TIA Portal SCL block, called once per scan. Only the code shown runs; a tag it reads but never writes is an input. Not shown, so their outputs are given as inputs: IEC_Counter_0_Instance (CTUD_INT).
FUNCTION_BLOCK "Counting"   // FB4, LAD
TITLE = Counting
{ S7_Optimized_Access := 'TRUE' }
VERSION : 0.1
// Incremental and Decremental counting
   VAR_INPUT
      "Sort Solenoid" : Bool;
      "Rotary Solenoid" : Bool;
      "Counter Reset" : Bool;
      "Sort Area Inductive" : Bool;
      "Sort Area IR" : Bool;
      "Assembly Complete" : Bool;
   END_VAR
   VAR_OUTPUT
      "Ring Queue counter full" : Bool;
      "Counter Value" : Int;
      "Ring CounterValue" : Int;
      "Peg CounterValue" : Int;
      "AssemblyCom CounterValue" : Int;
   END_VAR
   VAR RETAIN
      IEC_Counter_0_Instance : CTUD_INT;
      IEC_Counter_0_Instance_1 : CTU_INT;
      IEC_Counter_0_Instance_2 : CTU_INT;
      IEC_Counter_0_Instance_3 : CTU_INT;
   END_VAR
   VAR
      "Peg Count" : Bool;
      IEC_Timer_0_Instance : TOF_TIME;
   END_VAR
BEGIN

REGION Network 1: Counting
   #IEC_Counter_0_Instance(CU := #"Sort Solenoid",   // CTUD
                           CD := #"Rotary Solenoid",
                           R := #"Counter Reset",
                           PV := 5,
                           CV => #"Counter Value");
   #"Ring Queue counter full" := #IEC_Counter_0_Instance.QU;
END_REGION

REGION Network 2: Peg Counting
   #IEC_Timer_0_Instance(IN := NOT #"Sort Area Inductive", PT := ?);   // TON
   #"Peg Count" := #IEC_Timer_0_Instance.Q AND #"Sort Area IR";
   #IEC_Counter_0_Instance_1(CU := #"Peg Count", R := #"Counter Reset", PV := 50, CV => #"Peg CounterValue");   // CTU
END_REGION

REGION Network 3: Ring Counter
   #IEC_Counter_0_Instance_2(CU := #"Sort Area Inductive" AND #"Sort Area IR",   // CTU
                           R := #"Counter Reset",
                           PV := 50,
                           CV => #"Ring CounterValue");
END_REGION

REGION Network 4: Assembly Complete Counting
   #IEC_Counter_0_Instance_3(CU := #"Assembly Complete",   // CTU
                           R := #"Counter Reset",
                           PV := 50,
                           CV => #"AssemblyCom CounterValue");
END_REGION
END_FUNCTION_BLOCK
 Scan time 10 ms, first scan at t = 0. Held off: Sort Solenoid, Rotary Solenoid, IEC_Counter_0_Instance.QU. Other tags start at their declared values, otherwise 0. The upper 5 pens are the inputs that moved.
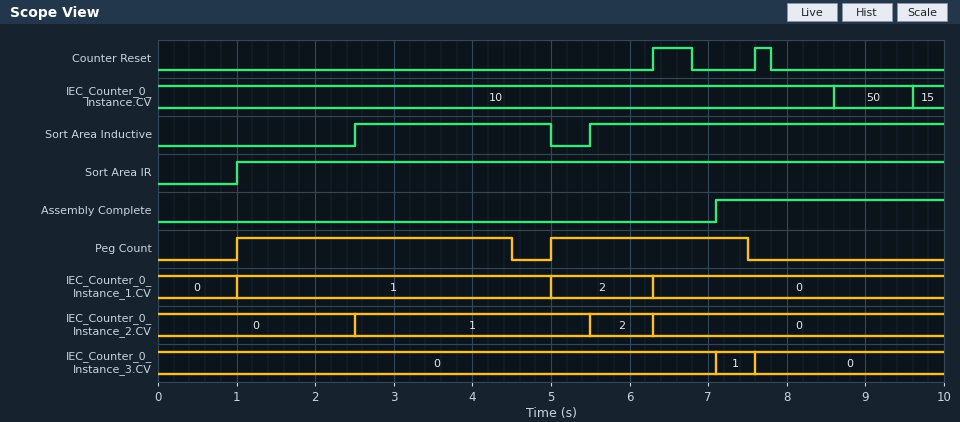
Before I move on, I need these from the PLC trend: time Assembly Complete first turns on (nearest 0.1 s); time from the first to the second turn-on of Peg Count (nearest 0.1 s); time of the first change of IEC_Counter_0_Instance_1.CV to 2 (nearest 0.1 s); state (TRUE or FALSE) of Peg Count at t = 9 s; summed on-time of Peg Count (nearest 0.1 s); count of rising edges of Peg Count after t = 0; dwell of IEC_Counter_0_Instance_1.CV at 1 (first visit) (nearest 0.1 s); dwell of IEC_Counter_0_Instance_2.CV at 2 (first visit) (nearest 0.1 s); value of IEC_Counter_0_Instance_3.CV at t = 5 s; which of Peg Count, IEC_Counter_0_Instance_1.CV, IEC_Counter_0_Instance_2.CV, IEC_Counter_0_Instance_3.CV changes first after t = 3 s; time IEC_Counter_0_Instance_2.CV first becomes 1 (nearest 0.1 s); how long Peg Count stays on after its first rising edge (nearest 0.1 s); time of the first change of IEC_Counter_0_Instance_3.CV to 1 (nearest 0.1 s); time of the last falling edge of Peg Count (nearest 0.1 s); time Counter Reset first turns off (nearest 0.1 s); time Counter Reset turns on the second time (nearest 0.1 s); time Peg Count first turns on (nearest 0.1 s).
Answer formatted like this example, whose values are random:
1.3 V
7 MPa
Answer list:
7.1 s
4.0 s
5.0 s
FALSE
6.0 s
2
4.0 s
0.8 s
0
Peg Count
2.5 s
3.5 s
7.1 s
7.5 s
6.8 s
7.6 s
1.0 s
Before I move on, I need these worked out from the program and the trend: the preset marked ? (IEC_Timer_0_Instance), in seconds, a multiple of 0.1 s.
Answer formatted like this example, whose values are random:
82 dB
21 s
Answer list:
2.0 s
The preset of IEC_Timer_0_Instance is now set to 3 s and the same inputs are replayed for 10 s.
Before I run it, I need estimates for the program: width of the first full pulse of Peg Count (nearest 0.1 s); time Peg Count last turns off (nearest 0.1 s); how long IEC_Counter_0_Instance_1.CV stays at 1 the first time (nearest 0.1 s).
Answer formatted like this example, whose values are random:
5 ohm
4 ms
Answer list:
7.5 s
8.5 s
5.3 s
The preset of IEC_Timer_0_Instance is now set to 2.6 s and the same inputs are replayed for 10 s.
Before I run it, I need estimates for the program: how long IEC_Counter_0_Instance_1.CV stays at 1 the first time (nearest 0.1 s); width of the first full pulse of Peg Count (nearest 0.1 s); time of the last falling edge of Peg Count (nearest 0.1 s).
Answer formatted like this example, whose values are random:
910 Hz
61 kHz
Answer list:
5.3 s
7.1 s
8.1 s
